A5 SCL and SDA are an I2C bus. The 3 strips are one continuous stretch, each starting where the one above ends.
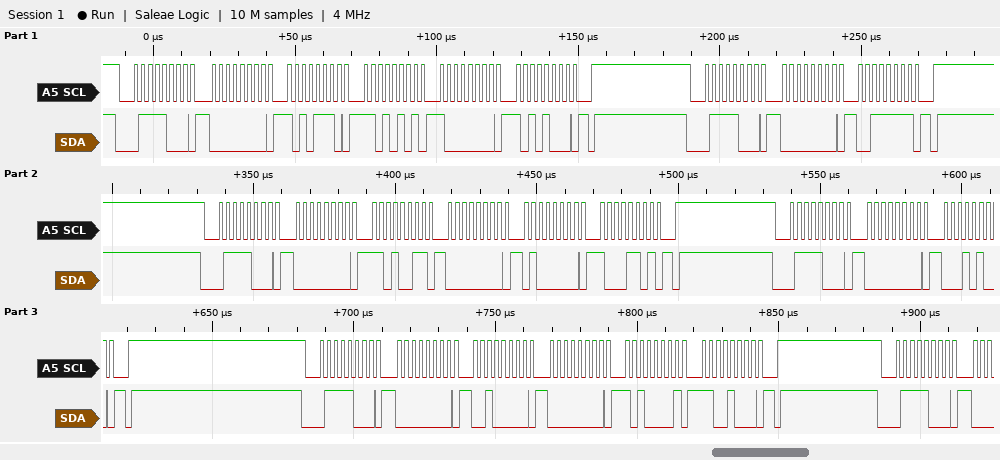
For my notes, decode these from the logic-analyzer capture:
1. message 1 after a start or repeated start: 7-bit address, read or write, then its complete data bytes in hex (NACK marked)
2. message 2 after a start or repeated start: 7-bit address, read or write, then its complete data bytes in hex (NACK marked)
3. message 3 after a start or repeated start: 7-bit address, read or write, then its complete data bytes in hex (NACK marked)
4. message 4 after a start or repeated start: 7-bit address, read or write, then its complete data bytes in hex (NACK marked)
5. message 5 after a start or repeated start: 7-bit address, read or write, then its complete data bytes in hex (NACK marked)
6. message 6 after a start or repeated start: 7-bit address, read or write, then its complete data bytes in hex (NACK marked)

0x3C write: 00 AE D5 80 A8
0x3C write: 00 3F
0x3C write: 00 D3 00 40 8D
0x3C write: 00 14
0x3C write: 00 20 00 A1 C8
0x3C write
